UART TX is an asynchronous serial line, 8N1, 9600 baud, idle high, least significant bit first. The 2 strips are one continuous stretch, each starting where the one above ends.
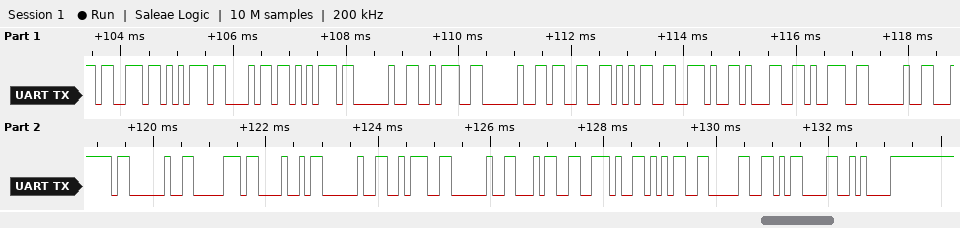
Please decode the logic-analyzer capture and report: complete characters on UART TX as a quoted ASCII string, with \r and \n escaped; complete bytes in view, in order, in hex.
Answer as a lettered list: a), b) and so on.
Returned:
a) "suhu : 35.19 | pH : 4.50\r\n"
b) 73 75 68 75 20 3A 20 33 35 2E 31 39 20 7C 20 70 48 20 3A 20 34 2E 35 30 0D 0A
